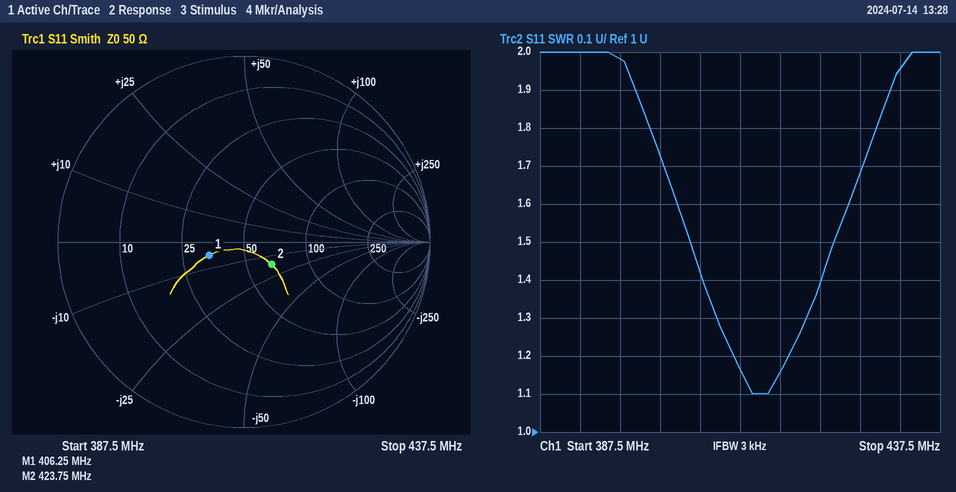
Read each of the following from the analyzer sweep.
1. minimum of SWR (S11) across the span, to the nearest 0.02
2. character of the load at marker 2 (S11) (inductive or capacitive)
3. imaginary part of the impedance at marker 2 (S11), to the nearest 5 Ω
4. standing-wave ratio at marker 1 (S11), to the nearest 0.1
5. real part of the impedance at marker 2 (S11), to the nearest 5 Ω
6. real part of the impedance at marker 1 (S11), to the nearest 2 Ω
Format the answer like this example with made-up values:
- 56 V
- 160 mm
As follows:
- 1.10
- capacitive
- -15 Ω
- 1.5
- 65 Ω
- 34 Ω
